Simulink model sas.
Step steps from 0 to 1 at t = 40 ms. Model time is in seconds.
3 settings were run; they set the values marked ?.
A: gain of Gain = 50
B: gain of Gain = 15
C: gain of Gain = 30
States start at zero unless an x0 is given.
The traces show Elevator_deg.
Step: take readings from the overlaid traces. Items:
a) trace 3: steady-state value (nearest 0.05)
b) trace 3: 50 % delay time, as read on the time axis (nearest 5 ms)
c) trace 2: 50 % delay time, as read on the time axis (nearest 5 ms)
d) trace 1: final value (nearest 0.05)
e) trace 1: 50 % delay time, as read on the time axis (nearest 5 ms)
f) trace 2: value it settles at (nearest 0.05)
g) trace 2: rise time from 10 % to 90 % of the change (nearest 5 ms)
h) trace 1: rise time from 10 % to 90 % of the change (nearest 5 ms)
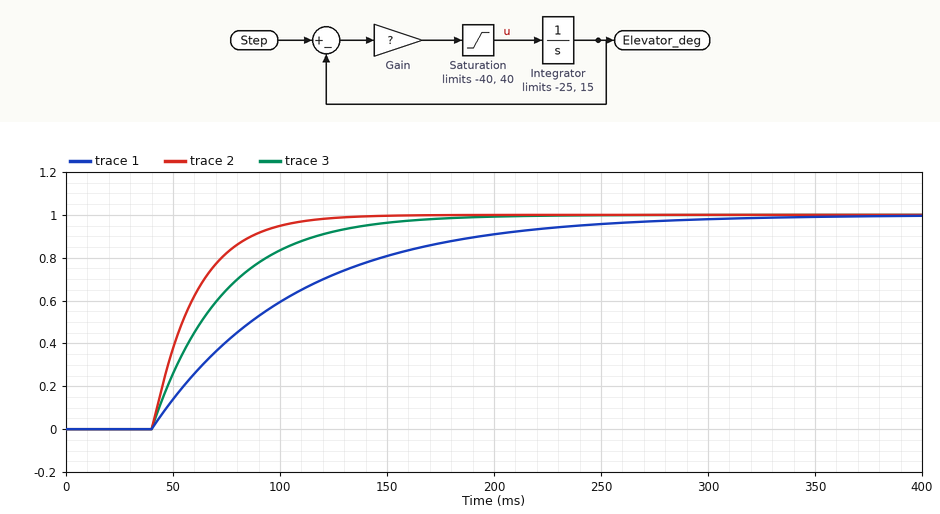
1.00
65 ms
55 ms
1.00
85 ms
1.00
45 ms
145 ms
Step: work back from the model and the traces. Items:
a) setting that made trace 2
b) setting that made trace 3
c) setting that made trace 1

A
C
B
